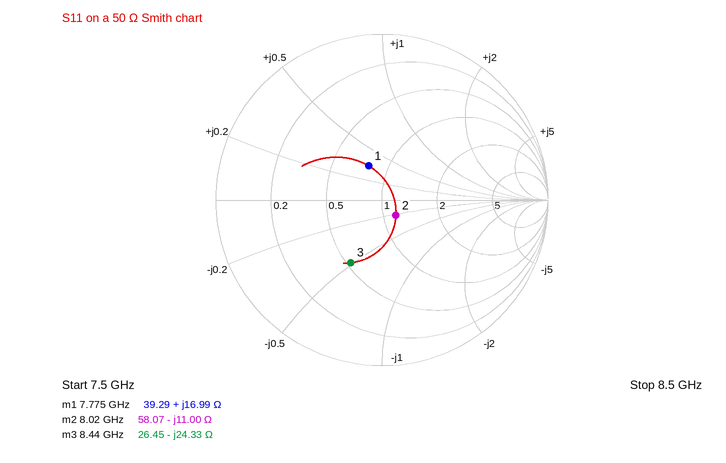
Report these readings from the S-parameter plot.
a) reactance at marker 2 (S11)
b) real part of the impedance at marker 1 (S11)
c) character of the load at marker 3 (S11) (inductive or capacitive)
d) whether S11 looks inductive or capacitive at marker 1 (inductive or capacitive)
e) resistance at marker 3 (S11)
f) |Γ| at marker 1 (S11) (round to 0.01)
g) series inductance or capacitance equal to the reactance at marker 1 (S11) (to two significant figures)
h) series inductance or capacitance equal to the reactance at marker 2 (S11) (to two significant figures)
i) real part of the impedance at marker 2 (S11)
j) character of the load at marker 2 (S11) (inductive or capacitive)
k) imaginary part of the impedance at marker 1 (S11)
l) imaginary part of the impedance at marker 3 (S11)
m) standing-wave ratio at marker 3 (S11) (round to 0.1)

-11.00 Ω
39.29 Ω
capacitive
inductive
26.45 Ω
0.22
350 pH
1.8 pF
58.07 Ω
capacitive
+16.99 Ω
-24.33 Ω
2.5
